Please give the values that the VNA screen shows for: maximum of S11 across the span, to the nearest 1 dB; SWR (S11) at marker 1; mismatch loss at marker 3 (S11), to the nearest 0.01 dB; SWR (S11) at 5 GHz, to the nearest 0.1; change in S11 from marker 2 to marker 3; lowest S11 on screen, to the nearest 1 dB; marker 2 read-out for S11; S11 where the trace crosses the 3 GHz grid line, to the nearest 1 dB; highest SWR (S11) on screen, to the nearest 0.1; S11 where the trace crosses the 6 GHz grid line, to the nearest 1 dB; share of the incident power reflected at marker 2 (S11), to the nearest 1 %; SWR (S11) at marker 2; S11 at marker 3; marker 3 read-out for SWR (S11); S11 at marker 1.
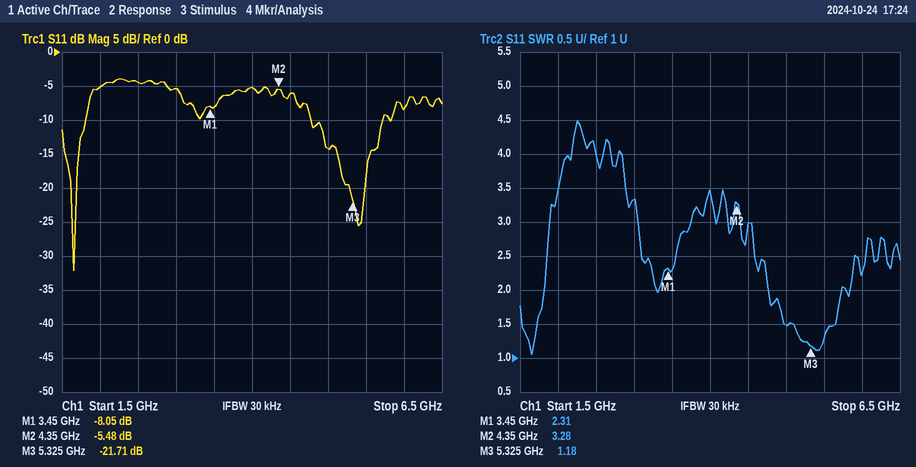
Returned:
-4 dB
2.31
0.03 dB
1.5
-16.23 dB
-32 dB
-5.48 dB
-5 dB
4.5
-8 dB
28 %
3.28
-21.71 dB
1.18
-8.05 dB
